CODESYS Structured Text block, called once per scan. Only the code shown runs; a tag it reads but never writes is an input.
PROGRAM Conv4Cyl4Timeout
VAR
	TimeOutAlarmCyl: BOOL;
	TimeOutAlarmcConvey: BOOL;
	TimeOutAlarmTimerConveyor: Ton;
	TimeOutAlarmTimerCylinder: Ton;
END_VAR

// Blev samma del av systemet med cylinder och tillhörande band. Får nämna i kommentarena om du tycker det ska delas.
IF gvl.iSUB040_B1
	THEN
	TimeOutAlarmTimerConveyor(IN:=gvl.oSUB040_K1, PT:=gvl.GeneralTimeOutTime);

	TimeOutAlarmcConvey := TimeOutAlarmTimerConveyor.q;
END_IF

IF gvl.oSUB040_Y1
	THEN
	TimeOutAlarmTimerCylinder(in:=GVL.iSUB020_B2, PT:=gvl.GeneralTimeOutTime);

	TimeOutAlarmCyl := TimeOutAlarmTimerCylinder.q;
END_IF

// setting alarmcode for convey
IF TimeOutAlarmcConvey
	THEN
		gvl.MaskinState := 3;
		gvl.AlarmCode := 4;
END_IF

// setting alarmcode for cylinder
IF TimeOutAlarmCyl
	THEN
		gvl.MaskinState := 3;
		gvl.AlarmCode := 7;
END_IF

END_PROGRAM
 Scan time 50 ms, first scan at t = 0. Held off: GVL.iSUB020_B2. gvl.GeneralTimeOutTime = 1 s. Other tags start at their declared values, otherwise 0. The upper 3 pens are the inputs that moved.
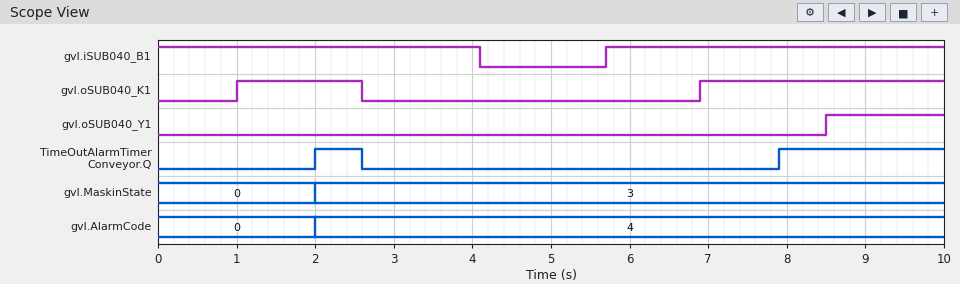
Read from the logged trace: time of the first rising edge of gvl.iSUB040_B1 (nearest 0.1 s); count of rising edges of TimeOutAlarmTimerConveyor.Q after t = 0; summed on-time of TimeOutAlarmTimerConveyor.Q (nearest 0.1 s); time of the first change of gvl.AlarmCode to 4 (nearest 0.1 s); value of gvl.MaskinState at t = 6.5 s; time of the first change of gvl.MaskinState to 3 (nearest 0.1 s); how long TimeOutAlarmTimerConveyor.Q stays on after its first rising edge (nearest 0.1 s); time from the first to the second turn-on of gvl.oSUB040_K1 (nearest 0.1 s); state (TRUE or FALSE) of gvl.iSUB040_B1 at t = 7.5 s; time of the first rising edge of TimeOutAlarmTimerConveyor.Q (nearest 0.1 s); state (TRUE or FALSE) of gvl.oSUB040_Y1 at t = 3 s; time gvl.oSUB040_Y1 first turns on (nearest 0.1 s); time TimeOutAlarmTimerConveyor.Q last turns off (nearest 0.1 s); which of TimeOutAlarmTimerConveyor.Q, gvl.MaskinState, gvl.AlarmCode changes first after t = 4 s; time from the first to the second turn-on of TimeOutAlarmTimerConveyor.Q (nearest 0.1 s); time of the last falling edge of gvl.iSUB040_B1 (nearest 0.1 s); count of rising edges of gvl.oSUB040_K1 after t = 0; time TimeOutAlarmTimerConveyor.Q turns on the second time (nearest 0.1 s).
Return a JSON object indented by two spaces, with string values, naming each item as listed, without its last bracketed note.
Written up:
{
  "time of the first rising edge of gvl.iSUB040_B1": "5.7 s",
  "count of rising edges of TimeOutAlarmTimerConveyor.Q after t = 0": "2",
  "summed on-time of TimeOutAlarmTimerConveyor.Q": "2.7 s",
  "time of the first change of gvl.AlarmCode to 4": "2.0 s",
  "value of gvl.MaskinState at t = 6.5 s": "3",
  "time of the first change of gvl.MaskinState to 3": "2.0 s",
  "how long TimeOutAlarmTimerConveyor.Q stays on after its first rising edge": "0.6 s",
  "time from the first to the second turn-on of gvl.oSUB040_K1": "5.9 s",
  "state (TRUE or FALSE) of gvl.iSUB040_B1 at t = 7.5 s": "TRUE",
  "time of the first rising edge of TimeOutAlarmTimerConveyor.Q": "2.0 s",
  "state (TRUE or FALSE) of gvl.oSUB040_Y1 at t = 3 s": "FALSE",
  "time gvl.oSUB040_Y1 first turns on": "8.5 s",
  "time TimeOutAlarmTimerConveyor.Q last turns off": "2.6 s",
  "which of TimeOutAlarmTimerConveyor.Q, gvl.MaskinState, gvl.AlarmCode changes first after t = 4 s": "TimeOutAlarmTimerConveyor.Q",
  "time from the first to the second turn-on of TimeOutAlarmTimerConveyor.Q": "5.9 s",
  "time of the last falling edge of gvl.iSUB040_B1": "4.1 s",
  "count of rising edges of gvl.oSUB040_K1 after t = 0": "2",
  "time TimeOutAlarmTimerConveyor.Q turns on the second time": "7.9 s"
}
